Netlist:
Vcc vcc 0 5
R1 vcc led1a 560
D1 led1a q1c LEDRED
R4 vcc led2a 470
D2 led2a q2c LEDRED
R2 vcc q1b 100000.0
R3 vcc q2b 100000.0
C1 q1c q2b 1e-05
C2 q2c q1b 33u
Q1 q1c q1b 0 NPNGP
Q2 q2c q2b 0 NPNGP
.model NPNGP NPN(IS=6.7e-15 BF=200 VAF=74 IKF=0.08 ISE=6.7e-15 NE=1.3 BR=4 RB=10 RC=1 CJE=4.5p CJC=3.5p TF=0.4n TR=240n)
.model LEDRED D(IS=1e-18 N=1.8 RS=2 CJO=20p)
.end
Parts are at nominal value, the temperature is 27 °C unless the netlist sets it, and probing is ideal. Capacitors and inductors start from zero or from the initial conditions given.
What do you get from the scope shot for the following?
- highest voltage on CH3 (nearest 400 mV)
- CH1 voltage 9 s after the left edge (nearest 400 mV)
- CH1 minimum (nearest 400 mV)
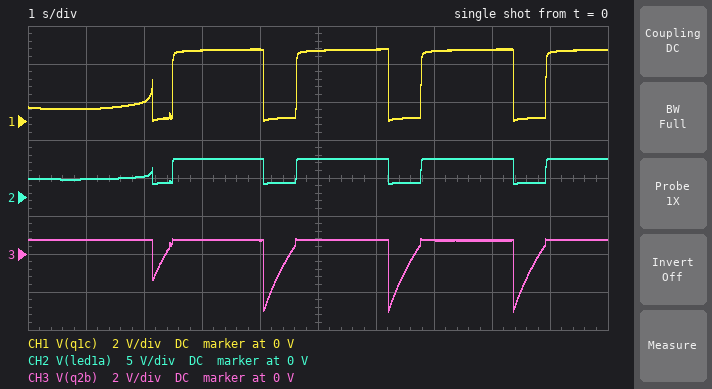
800 mV
3.6 V
0 V
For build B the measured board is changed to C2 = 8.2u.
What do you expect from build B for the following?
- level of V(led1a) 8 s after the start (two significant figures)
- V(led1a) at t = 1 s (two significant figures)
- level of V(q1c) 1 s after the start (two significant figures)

1.9 V
5.0 V
3.7 V
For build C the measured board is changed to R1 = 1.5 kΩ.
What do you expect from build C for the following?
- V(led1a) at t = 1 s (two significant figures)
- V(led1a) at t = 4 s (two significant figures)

5.0 V
5.0 V
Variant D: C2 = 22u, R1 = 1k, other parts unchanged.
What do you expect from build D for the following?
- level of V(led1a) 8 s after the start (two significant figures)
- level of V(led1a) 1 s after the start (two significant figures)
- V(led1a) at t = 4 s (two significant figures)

5.0 V
5.0 V
1.8 V
